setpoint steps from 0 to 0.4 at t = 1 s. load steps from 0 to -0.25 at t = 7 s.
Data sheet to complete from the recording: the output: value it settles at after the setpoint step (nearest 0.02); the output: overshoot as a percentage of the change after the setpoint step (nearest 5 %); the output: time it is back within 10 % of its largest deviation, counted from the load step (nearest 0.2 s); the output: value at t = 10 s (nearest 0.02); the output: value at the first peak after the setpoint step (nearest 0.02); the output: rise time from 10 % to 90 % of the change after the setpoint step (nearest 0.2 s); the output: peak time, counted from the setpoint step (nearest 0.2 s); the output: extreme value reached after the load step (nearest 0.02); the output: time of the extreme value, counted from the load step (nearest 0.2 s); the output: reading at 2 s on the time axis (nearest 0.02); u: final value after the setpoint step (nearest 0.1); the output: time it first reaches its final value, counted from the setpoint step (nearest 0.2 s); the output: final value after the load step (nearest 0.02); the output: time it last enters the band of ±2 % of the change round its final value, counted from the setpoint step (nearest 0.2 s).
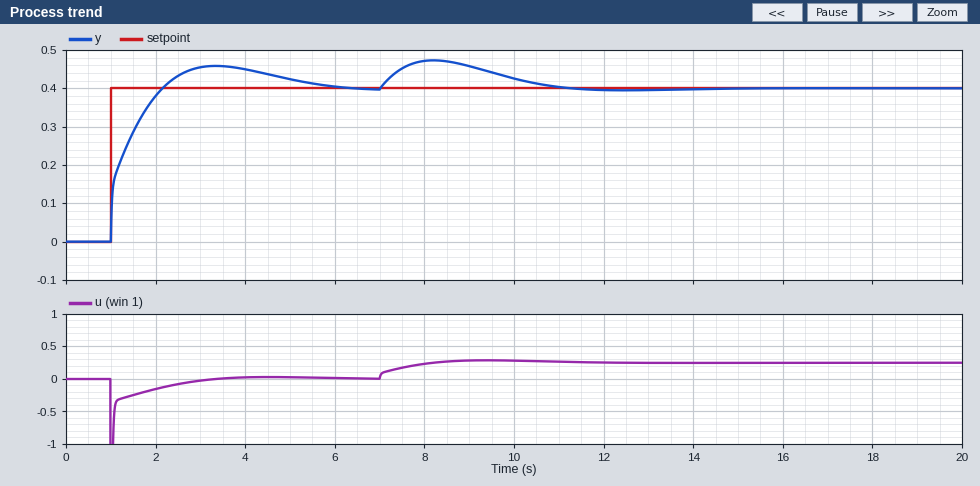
0.40
15 %
3.8 s
0.42
0.46
0.8 s
2.4 s
0.48
1.2 s
0.38
0.0
1.2 s
0.40
4.8 s
